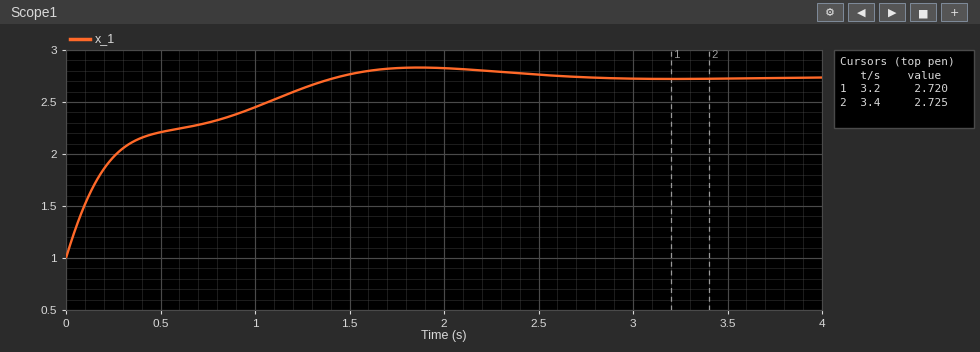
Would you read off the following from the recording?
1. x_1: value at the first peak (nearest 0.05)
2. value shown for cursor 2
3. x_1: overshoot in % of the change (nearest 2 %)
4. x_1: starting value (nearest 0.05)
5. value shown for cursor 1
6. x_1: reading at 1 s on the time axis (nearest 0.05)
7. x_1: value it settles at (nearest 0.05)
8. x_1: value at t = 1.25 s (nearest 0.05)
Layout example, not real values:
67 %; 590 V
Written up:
2.85; 2.725; 6 %; 1.00; 2.720; 2.45; 2.75; 2.65
